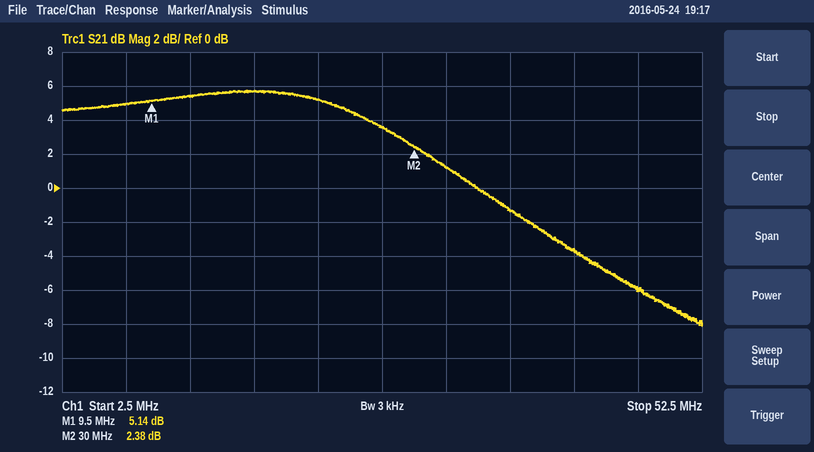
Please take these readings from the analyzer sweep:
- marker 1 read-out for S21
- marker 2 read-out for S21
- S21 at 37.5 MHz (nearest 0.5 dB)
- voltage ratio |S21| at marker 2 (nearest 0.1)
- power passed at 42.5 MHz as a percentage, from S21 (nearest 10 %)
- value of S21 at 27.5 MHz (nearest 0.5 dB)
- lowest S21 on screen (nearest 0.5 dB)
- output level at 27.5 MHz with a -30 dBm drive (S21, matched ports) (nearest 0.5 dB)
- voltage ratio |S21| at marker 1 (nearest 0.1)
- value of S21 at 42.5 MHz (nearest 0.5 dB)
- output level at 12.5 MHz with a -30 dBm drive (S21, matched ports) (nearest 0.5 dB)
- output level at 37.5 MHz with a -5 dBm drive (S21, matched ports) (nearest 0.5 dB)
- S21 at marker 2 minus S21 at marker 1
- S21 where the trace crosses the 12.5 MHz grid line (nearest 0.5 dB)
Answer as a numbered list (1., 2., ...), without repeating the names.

1. 5.14 dB
2. 2.38 dB
3. -1.5 dB
4. 1.3
5. 40 %
6. 3.5 dB
7. -8.0 dB
8. -26.5 dBm
9. 1.8
10. -3.5 dB
11. -24.5 dBm
12. -6.5 dBm
13. -2.76 dB
14. 5.5 dB
